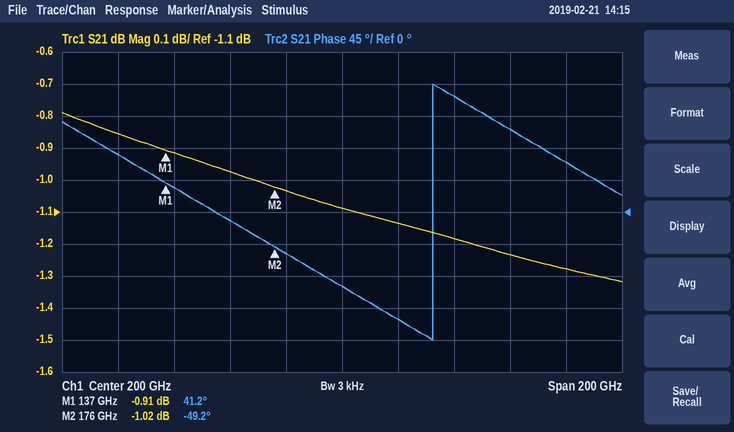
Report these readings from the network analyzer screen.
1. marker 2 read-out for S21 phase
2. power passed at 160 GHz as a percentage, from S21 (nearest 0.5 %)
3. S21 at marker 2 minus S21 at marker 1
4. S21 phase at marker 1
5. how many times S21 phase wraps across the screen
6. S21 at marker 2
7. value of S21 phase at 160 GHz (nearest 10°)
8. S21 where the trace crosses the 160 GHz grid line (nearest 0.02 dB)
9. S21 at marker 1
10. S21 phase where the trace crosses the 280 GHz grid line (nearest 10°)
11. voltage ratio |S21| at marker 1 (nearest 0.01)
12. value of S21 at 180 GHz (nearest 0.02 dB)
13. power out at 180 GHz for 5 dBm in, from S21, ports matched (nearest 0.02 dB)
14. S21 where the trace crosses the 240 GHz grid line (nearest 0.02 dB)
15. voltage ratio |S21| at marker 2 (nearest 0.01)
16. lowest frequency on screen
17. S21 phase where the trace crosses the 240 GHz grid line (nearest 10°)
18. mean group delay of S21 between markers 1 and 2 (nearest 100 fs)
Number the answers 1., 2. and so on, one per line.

1. -49.2°
2. 80.0 %
3. -0.11 dB
4. 41.2°
5. 1
6. -1.02 dB
7. -10°
8. -0.98 dB
9. -0.91 dB
10. 70°
11. 0.90
12. -1.04 dB
13. 3.96 dBm
14. -1.18 dB
15. 0.89
16. 100 GHz
17. 160°
18. 6.4 ps
